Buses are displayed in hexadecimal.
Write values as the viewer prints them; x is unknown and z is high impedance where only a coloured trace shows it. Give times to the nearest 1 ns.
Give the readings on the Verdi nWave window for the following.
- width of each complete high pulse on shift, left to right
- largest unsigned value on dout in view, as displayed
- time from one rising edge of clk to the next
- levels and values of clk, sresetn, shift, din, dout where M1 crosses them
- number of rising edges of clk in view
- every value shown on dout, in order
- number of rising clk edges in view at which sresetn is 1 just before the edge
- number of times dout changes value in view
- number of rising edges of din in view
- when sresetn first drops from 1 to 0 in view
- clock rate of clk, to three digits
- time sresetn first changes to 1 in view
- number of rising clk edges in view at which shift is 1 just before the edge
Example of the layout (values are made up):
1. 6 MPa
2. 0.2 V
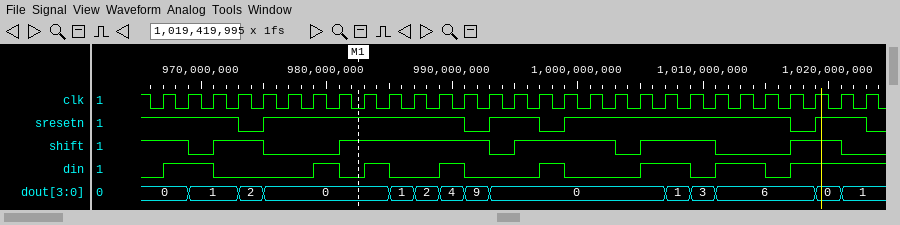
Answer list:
1. 4 ns, 12 ns, 8 ns, 6 ns, 4 ns
2. 9
3. 2 ns
4. clk=0, sresetn=1, shift=1, din=0, dout=0
5. 29
6. 0, 1, 2, 0, 1, 2, 4, 9, 0, 1, 3, 6, 0, 1
7. 25
8. 13
9. 8
10. 973 ns
11. 500 MHz
12. 975 ns
13. 19
